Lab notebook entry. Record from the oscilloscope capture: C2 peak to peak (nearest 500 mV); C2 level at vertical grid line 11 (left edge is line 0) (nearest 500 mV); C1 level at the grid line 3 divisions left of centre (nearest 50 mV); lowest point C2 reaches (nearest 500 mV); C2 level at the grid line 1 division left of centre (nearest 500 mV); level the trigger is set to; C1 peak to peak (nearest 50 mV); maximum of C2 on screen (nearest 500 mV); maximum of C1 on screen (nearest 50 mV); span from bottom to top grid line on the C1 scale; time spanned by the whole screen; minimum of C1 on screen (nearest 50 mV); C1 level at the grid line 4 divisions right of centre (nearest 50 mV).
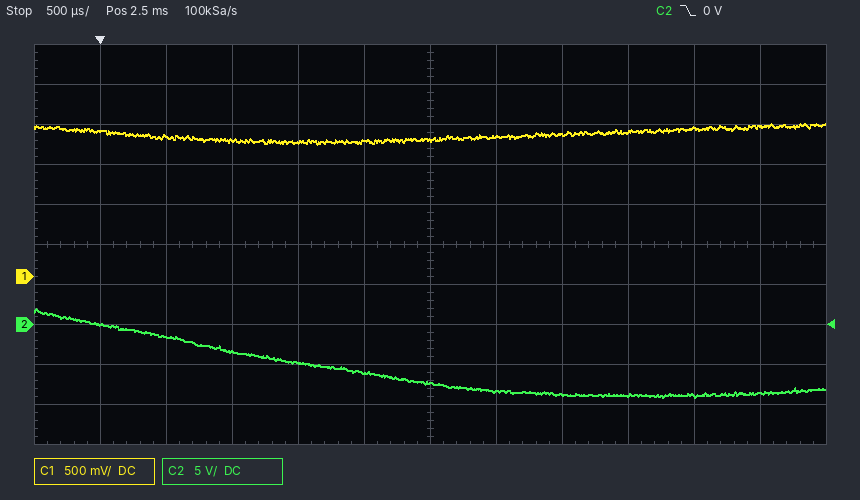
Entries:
11.0 V
-8.5 V
1.70 V
-9.0 V
-6.0 V
0 V
250 mV
2.0 V
1.90 V
5 V
6 ms
1.65 V
1.85 V
